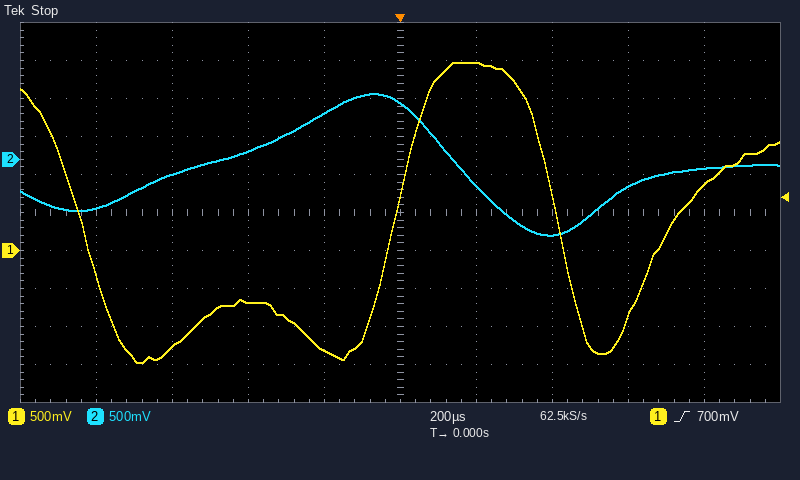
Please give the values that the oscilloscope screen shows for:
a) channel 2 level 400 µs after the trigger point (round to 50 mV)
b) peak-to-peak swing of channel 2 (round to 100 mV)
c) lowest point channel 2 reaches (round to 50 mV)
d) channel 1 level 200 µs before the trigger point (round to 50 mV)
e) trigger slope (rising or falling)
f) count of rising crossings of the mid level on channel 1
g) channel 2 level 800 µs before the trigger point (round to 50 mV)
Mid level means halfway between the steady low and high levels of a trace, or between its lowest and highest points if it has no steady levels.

-1.00 V
1.90 V
-1.00 V
-1.30 V
rising
2
-650 mV
